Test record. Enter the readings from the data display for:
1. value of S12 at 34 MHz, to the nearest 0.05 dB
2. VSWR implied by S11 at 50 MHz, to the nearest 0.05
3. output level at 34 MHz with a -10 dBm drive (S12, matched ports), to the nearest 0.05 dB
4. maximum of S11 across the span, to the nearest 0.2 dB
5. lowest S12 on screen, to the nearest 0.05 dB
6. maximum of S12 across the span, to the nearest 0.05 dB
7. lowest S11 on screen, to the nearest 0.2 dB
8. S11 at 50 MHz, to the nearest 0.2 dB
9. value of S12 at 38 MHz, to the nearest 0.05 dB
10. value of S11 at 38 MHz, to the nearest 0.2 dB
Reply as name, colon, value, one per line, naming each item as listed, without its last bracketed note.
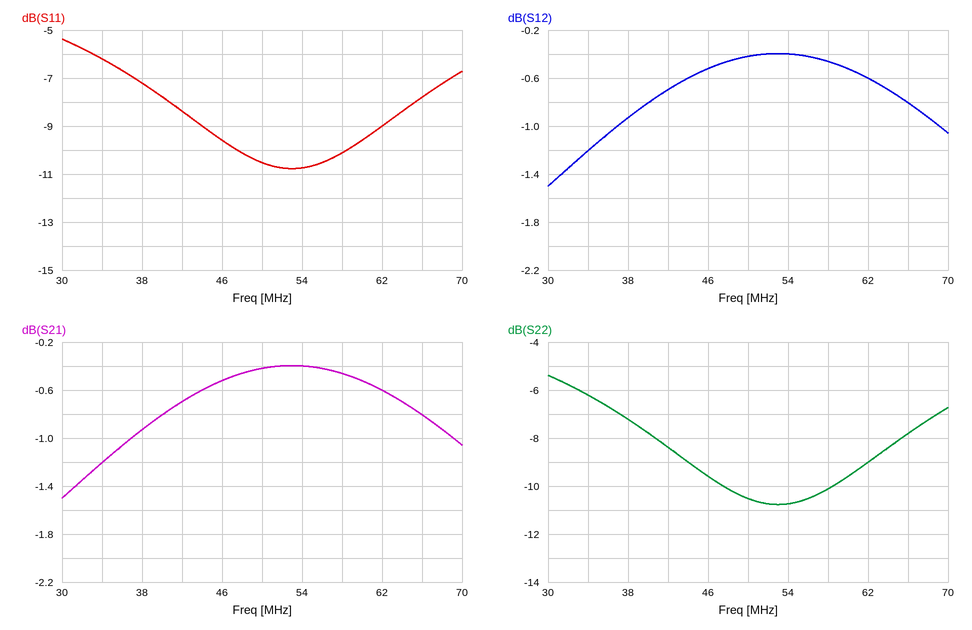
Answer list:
value of S12 at 34 MHz, to the nearest 0.05 dB: -1.20 dB
VSWR implied by S11 at 50 MHz, to the nearest 0.05: 1.85
output level at 34 MHz with a -10 dBm drive (S12, matched ports), to the nearest 0.05 dB: -11.20 dBm
maximum of S11 across the span, to the nearest 0.2 dB: -5.4 dB
lowest S12 on screen, to the nearest 0.05 dB: -1.50 dB
maximum of S12 across the span, to the nearest 0.05 dB: -0.40 dB
lowest S11 on screen, to the nearest 0.2 dB: -10.8 dB
S11 at 50 MHz, to the nearest 0.2 dB: -10.6 dB
value of S12 at 38 MHz, to the nearest 0.05 dB: -0.95 dB
value of S11 at 38 MHz, to the nearest 0.2 dB: -7.2 dB
